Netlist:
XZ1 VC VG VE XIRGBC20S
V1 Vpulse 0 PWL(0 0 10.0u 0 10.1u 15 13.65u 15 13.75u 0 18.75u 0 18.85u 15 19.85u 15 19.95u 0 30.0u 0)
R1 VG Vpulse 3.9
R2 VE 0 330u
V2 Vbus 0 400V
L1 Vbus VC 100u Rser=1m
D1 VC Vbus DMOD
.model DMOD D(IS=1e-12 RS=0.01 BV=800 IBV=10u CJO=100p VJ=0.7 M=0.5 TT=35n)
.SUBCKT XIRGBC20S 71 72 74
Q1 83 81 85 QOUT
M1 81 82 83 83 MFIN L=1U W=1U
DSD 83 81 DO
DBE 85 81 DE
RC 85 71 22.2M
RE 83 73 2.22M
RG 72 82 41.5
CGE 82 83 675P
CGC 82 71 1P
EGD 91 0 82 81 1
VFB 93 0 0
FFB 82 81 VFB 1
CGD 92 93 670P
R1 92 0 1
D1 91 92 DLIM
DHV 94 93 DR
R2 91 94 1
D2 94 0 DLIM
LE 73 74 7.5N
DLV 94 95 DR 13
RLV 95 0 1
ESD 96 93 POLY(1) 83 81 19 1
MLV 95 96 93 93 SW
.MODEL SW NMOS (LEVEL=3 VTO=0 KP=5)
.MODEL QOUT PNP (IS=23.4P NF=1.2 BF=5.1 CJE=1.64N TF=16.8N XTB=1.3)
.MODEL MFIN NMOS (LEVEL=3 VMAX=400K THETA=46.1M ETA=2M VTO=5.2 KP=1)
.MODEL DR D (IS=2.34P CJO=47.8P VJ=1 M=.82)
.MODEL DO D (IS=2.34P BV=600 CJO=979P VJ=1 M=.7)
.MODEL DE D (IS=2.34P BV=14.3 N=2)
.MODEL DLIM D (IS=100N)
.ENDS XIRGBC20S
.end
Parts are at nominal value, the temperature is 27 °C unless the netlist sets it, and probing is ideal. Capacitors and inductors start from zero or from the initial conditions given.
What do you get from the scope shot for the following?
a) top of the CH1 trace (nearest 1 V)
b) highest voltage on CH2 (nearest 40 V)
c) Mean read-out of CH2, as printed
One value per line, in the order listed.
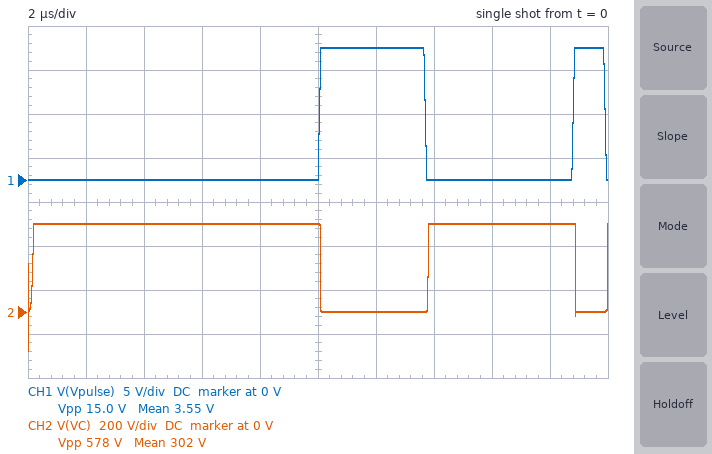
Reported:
15 V
400 V
302 V
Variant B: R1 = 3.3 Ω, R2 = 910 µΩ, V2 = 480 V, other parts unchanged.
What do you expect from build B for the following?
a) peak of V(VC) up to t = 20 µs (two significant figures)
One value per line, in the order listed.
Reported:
480 V
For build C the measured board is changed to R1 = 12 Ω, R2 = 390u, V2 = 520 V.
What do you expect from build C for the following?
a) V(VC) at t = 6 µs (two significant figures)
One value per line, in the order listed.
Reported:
520 V
